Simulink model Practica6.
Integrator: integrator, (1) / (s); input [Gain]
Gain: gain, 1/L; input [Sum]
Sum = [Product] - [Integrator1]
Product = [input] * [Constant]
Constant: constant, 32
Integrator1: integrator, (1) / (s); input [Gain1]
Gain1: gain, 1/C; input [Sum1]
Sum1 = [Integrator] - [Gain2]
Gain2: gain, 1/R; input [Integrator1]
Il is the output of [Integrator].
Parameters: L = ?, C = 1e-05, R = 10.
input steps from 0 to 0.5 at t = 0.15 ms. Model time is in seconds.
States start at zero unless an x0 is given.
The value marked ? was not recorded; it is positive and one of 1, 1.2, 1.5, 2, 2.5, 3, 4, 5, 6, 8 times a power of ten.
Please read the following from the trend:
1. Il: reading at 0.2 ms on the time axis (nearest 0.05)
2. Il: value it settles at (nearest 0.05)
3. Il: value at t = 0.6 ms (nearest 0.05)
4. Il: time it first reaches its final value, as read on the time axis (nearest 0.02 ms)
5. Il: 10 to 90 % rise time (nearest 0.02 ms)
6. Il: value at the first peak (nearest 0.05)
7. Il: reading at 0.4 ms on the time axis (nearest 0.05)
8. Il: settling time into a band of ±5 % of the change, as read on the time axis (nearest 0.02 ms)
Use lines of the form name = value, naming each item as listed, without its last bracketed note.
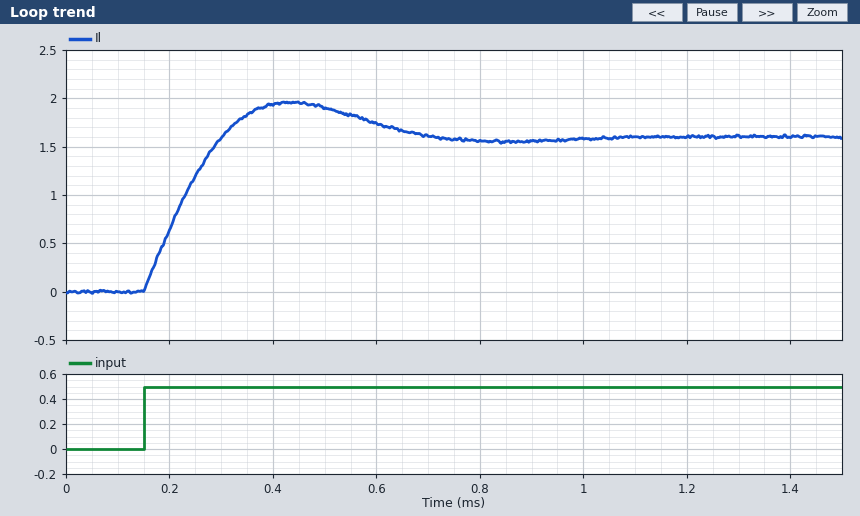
Il: reading at 0.2 ms on the time axis = 0.65
Il: value it settles at = 1.60
Il: value at t = 0.6 ms = 1.75
Il: time it first reaches its final value, as read on the time axis = 0.30 ms
Il: 10 to 90 % rise time = 0.12 ms
Il: value at the first peak = 1.95
Il: reading at 0.4 ms on the time axis = 1.95
Il: settling time into a band of ±5 % of the change, as read on the time axis = 0.64 ms
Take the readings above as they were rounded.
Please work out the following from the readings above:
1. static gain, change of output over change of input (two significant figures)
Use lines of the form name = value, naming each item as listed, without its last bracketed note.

static gain, change of output over change of input = 3.2
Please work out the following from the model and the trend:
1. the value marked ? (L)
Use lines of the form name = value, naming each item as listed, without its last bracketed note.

the value marked ? = 0.0012
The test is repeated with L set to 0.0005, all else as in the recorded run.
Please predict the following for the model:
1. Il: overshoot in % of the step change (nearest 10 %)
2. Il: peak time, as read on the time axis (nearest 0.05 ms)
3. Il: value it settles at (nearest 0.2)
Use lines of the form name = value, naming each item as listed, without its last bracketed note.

Il: overshoot in % of the step change = 70 %
Il: peak time, as read on the time axis = 0.30 ms
Il: value it settles at = 1.6
